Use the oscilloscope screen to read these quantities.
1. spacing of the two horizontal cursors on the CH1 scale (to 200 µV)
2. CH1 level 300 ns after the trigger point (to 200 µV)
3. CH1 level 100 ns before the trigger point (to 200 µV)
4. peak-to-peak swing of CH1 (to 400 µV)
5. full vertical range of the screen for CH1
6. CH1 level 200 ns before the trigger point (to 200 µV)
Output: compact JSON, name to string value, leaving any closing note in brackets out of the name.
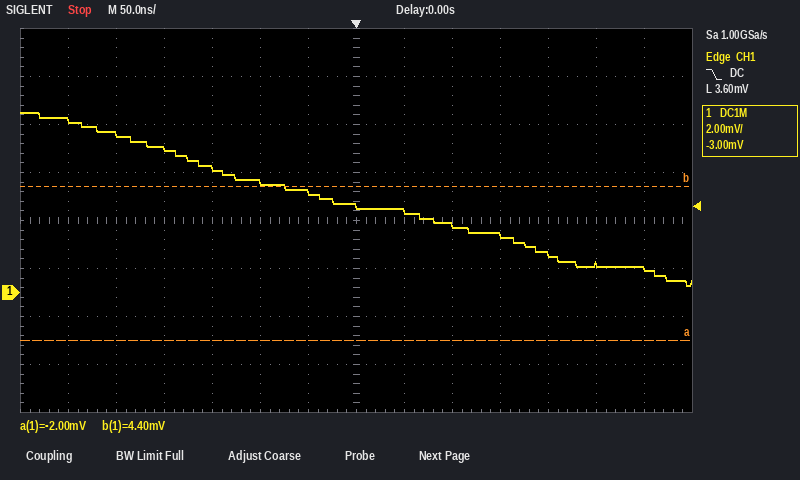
{"spacing of the two horizontal cursors on the CH1 scale": "6.4 mV", "CH1 level 300 ns after the trigger point": "1.0 mV", "CH1 level 100 ns before the trigger point": "4.6 mV", "peak-to-peak swing of CH1": "7.2 mV", "full vertical range of the screen for CH1": "16 mV", "CH1 level 200 ns before the trigger point": "6.0 mV"}
